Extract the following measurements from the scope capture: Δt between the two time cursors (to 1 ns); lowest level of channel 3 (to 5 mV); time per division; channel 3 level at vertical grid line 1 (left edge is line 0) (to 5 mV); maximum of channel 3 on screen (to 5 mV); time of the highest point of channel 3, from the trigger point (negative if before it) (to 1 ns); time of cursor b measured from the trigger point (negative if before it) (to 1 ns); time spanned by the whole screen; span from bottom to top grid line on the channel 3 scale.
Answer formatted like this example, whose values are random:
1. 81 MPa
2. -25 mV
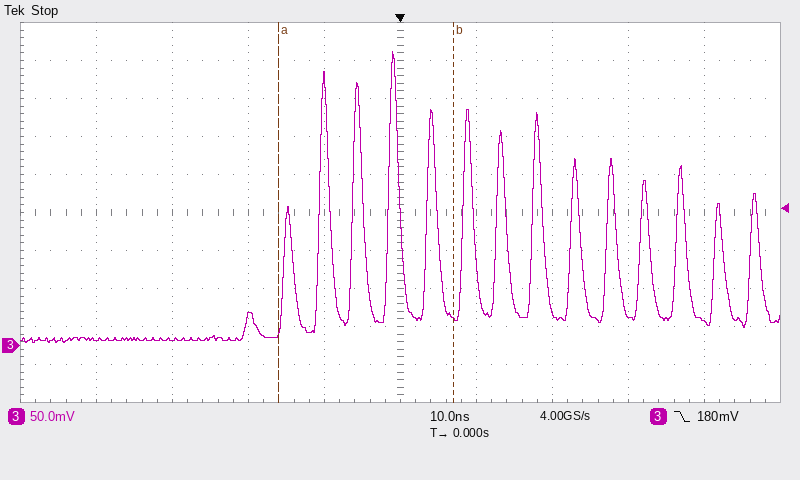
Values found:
1. 23 ns
2. 5 mV
3. 10 ns
4. 10 mV
5. 385 mV
6. -1 ns
7. +7 ns
8. 100 ns
9. 500 mV
